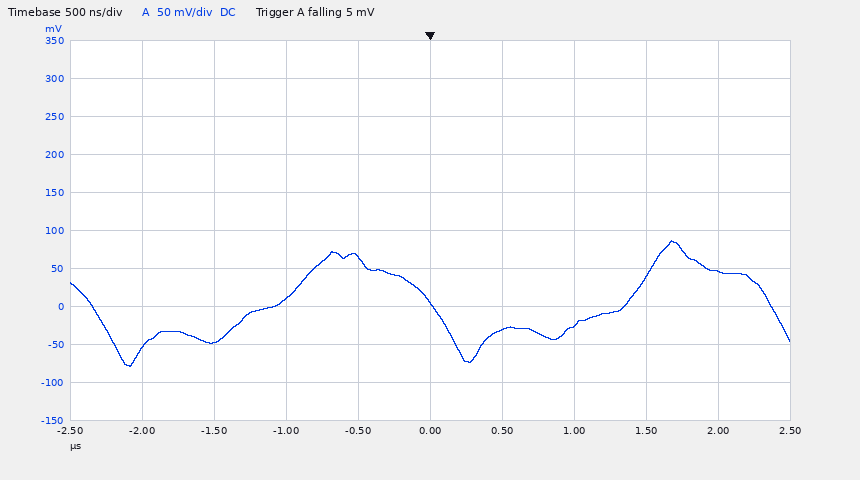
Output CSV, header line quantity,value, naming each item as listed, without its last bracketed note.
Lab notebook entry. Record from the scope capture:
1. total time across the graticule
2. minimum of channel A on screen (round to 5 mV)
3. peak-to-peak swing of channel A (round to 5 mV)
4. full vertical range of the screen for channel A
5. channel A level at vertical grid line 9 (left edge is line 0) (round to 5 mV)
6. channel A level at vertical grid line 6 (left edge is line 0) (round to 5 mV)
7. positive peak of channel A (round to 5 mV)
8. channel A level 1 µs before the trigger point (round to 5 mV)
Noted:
quantity,value
total time across the graticule,5 µs
minimum of channel A on screen,-80 mV
peak-to-peak swing of channel A,165 mV
full vertical range of the screen for channel A,500 mV
channel A level at vertical grid line 9 (left edge is line 0),45 mV
channel A level at vertical grid line 6 (left edge is line 0),-30 mV
positive peak of channel A,85 mV
channel A level 1 µs before the trigger point,10 mV
